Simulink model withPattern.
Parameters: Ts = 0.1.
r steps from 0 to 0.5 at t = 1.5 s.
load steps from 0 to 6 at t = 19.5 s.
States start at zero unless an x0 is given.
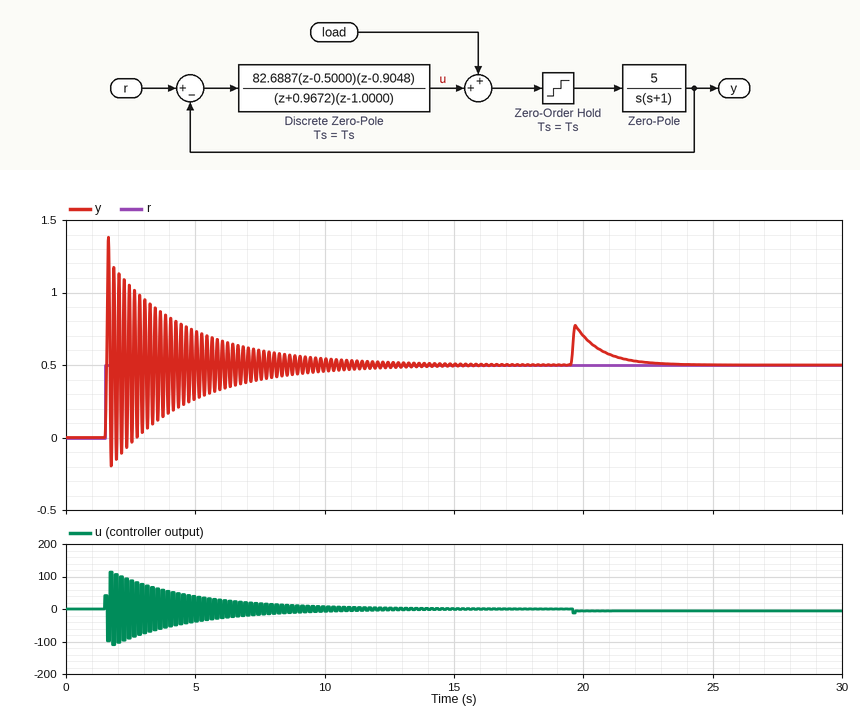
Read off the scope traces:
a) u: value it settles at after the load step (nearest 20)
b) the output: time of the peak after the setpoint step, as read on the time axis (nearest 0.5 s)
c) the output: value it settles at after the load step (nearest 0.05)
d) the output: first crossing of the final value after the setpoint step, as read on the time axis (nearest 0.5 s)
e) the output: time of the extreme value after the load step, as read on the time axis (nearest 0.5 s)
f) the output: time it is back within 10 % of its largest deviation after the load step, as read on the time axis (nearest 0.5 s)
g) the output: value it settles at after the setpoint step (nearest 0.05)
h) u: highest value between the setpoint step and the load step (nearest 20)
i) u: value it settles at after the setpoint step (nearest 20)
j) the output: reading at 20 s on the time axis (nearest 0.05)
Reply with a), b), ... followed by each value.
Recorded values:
a) 0
b) 1.5 s
c) 0.50
d) 1.5 s
e) 19.5 s
f) 22.0 s
g) 0.50
h) 120
i) 0
j) 0.70
